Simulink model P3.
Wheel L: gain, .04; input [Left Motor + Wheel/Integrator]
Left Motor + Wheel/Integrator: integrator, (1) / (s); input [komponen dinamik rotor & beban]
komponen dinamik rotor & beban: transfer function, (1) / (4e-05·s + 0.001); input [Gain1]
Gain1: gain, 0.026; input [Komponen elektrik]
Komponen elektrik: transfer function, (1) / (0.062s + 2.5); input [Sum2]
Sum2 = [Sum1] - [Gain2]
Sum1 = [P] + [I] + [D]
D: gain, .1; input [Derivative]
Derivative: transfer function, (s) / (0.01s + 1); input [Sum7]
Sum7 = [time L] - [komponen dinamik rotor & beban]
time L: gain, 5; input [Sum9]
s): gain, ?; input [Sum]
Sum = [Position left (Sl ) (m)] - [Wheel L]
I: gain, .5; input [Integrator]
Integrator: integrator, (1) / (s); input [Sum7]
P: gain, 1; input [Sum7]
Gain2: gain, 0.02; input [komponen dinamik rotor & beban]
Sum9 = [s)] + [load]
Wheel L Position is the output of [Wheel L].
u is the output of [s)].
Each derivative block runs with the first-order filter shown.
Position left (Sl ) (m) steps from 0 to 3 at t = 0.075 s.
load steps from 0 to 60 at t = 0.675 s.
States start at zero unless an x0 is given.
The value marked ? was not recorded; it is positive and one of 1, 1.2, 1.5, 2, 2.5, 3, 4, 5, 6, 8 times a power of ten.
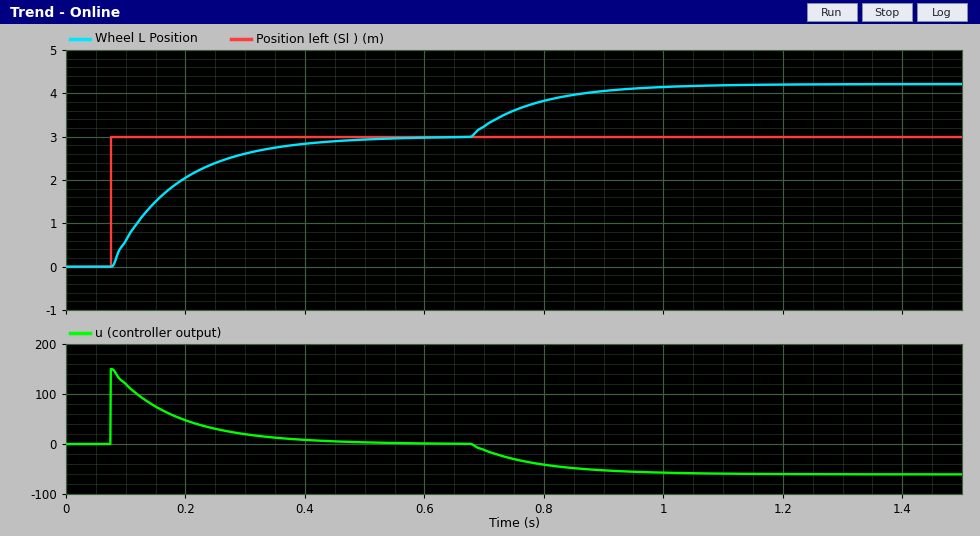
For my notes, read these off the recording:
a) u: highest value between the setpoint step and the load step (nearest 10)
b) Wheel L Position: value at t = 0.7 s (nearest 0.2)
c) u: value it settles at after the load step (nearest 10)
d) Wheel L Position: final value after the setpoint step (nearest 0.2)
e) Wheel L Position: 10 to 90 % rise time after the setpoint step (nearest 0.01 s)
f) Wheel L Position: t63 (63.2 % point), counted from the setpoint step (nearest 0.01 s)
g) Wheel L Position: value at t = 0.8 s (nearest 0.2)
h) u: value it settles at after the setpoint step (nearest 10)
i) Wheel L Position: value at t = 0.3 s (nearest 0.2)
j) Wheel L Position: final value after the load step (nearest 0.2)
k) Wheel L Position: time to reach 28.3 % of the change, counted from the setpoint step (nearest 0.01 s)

150
3.2
-60
3.0
0.24 s
0.11 s
3.8
0
2.6
4.2
0.04 s
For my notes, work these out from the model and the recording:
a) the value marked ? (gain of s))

50
